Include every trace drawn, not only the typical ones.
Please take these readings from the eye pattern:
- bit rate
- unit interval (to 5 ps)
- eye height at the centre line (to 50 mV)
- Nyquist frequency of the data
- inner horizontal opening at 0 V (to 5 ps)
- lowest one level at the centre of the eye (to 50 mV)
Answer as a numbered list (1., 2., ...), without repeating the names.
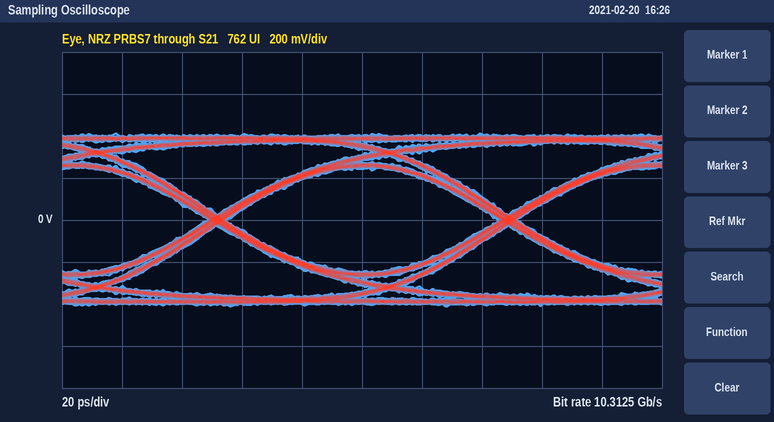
1. 10.3125 Gb/s
2. 95 ps
3. 500 mV
4. 5.15625 GHz
5. 90 ps
6. 250 mV
